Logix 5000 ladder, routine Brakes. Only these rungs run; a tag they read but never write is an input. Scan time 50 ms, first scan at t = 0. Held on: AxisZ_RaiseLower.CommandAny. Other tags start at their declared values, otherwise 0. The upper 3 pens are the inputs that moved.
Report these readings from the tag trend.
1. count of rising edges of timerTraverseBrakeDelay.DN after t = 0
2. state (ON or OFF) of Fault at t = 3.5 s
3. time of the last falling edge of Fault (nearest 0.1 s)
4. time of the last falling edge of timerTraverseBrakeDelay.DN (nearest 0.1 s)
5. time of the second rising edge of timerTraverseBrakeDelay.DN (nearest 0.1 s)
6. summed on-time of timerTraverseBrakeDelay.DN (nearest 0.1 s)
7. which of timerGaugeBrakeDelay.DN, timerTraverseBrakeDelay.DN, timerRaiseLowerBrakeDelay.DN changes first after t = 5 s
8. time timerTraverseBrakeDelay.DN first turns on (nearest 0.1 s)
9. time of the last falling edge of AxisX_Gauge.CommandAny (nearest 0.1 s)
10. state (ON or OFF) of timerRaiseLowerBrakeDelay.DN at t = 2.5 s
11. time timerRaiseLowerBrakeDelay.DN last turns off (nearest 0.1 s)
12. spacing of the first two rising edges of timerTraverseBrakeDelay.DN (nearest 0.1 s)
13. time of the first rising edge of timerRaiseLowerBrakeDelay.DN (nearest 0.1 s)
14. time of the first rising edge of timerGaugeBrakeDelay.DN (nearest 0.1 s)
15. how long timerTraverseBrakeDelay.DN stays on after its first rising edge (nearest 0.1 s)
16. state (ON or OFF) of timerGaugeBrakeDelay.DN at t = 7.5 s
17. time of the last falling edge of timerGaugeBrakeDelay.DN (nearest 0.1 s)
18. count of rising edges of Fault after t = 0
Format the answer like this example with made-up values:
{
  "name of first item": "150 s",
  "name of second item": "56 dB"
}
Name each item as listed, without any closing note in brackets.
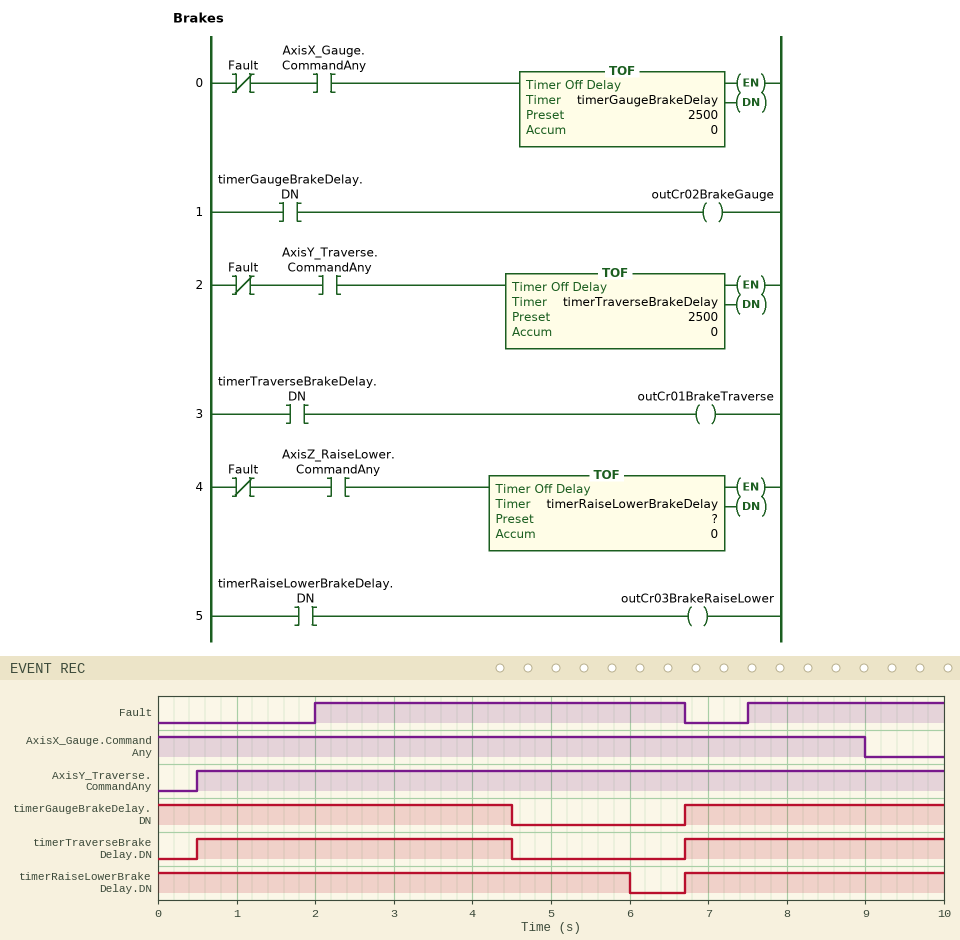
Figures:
{
  "count of rising edges of timerTraverseBrakeDelay.DN after t = 0": "2",
  "state (ON or OFF) of Fault at t = 3.5 s": "ON",
  "time of the last falling edge of Fault": "6.7 s",
  "time of the last falling edge of timerTraverseBrakeDelay.DN": "4.5 s",
  "time of the second rising edge of timerTraverseBrakeDelay.DN": "6.7 s",
  "summed on-time of timerTraverseBrakeDelay.DN": "7.3 s",
  "which of timerGaugeBrakeDelay.DN, timerTraverseBrakeDelay.DN, timerRaiseLowerBrakeDelay.DN changes first after t = 5 s": "timerRaiseLowerBrakeDelay.DN",
  "time timerTraverseBrakeDelay.DN first turns on": "0.5 s",
  "time of the last falling edge of AxisX_Gauge.CommandAny": "9.0 s",
  "state (ON or OFF) of timerRaiseLowerBrakeDelay.DN at t = 2.5 s": "ON",
  "time timerRaiseLowerBrakeDelay.DN last turns off": "6.0 s",
  "spacing of the first two rising edges of timerTraverseBrakeDelay.DN": "6.2 s",
  "time of the first rising edge of timerRaiseLowerBrakeDelay.DN": "6.7 s",
  "time of the first rising edge of timerGaugeBrakeDelay.DN": "6.7 s",
  "how long timerTraverseBrakeDelay.DN stays on after its first rising edge": "4.0 s",
  "state (ON or OFF) of timerGaugeBrakeDelay.DN at t = 7.5 s": "ON",
  "time of the last falling edge of timerGaugeBrakeDelay.DN": "4.5 s",
  "count of rising edges of Fault after t = 0": "2"
}
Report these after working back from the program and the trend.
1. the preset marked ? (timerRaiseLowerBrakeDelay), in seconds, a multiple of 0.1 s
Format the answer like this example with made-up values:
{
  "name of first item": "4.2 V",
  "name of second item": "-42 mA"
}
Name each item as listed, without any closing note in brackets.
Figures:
{
  "the preset marked ? (timerRaiseLowerBrakeDelay), in seconds, a multiple of 0.1 s": "4.0 s"
}
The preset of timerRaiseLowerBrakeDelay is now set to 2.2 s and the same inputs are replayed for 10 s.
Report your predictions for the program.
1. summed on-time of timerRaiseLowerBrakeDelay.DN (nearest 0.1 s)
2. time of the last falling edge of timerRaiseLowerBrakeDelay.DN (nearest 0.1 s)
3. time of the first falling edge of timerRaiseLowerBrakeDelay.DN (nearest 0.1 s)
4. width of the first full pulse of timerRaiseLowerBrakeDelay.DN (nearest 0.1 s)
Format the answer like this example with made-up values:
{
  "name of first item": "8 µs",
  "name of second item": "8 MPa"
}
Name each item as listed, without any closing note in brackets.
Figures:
{
  "summed on-time of timerRaiseLowerBrakeDelay.DN": "7.2 s",
  "time of the last falling edge of timerRaiseLowerBrakeDelay.DN": "9.7 s",
  "time of the first falling edge of timerRaiseLowerBrakeDelay.DN": "4.2 s",
  "width of the first full pulse of timerRaiseLowerBrakeDelay.DN": "3.0 s"
}
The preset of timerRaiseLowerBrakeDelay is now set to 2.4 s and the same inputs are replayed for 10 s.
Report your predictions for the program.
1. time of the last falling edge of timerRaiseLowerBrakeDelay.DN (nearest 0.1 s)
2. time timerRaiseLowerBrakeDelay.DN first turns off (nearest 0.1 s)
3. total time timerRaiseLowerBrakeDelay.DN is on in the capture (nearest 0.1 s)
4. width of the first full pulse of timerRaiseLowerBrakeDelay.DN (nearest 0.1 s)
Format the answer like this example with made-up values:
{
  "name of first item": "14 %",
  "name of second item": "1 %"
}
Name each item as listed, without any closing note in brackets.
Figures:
{
  "time of the last falling edge of timerRaiseLowerBrakeDelay.DN": "9.9 s",
  "time timerRaiseLowerBrakeDelay.DN first turns off": "4.4 s",
  "total time timerRaiseLowerBrakeDelay.DN is on in the capture": "7.6 s",
  "width of the first full pulse of timerRaiseLowerBrakeDelay.DN": "3.2 s"
}
